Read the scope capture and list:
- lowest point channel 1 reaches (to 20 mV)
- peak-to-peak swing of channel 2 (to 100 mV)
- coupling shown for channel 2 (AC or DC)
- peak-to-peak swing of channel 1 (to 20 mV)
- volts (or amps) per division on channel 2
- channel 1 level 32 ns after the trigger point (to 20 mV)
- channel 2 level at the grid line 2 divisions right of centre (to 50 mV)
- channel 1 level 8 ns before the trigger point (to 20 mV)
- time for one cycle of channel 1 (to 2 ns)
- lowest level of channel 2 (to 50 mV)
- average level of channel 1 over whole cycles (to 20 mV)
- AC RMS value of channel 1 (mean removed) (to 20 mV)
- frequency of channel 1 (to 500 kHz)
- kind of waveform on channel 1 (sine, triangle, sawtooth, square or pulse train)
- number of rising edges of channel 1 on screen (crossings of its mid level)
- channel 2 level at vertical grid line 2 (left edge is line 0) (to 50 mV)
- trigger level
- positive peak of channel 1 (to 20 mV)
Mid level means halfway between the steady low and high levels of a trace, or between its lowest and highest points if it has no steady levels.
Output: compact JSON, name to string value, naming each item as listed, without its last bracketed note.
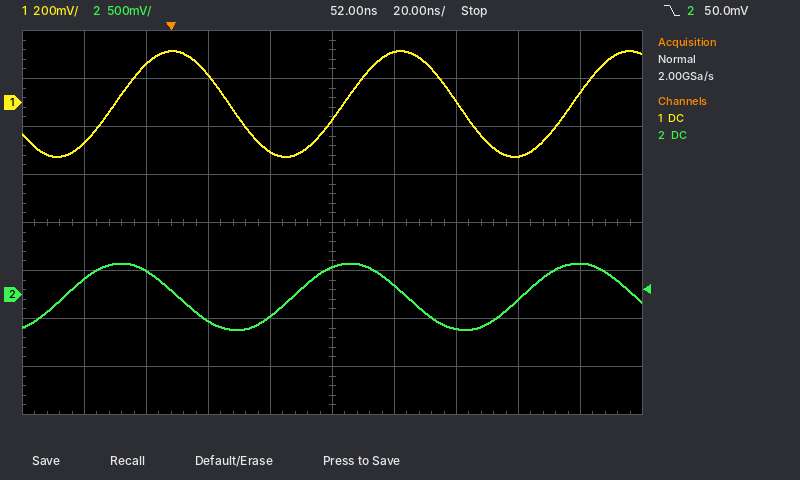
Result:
{"lowest point channel 1 reaches": "-220 mV", "peak-to-peak swing of channel 2": "700 mV", "coupling shown for channel 2": "DC", "peak-to-peak swing of channel 1": "440 mV", "volts (or amps) per division on channel 2": "500 mV", "channel 1 level 32 ns after the trigger point": "-200 mV", "channel 2 level at the grid line 2 divisions right of centre": "-350 mV", "channel 1 level 8 ns before the trigger point": "160 mV", "time for one cycle of channel 1": "74 ns", "lowest level of channel 2": "-350 mV", "average level of channel 1 over whole cycles": "0 mV", "AC RMS value of channel 1 (mean removed)": "160 mV", "frequency of channel 1": "13.5 MHz", "kind of waveform on channel 1": "sine", "number of rising edges of channel 1 on screen": "3", "channel 2 level at vertical grid line 2 (left edge is line 0)": "250 mV", "trigger level": "50.0 mV", "positive peak of channel 1": "220 mV"}
